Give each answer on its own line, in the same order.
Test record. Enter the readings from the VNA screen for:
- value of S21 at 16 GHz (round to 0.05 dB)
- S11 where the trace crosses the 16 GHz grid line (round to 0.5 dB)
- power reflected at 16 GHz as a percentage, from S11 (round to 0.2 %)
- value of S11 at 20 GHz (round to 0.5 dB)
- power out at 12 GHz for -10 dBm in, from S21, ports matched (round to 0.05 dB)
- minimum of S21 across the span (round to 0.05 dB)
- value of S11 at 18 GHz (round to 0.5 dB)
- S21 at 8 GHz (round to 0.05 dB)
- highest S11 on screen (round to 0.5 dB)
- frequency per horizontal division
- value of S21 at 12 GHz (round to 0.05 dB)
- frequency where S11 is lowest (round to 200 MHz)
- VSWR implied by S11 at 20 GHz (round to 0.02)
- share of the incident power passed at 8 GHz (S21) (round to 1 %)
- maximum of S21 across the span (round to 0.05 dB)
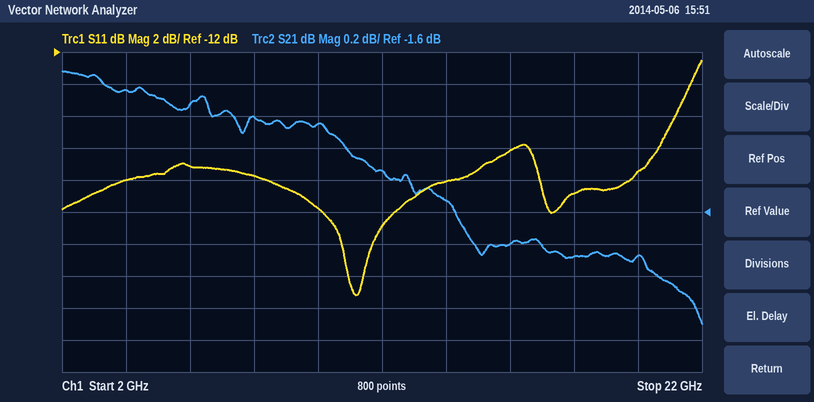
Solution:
-1.80 dB
-18.0 dB
1.6 %
-19.5 dB
-11.35 dBm
-2.30 dB
-21.0 dB
-1.00 dB
-12.5 dB
2 GHz
-1.35 dB
11.2 GHz
1.24
79 %
-0.70 dB
